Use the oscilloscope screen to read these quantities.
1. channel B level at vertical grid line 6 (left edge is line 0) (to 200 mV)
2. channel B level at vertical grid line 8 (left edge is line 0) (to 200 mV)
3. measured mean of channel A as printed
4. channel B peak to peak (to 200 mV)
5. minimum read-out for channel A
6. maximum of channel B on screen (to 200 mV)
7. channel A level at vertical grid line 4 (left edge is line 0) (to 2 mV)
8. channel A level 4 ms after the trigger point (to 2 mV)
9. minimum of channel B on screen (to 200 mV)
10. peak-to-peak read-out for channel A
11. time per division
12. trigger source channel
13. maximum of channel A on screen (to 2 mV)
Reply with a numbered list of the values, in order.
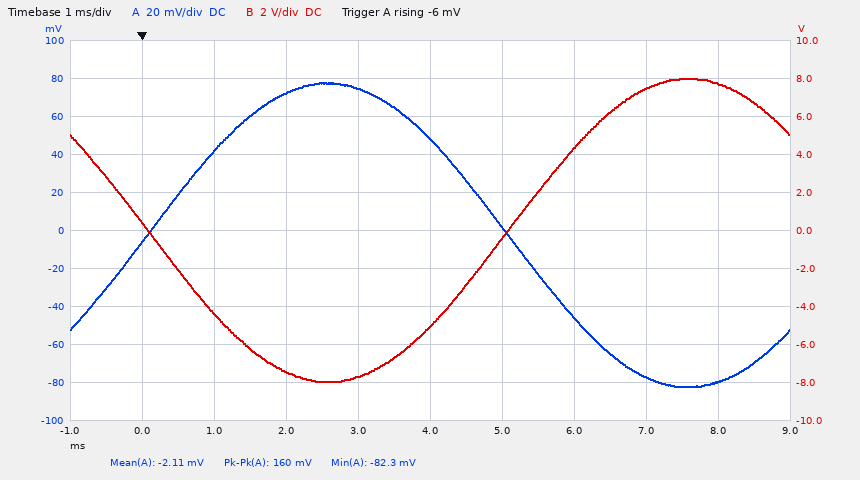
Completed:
1. -400 mV
2. 7.4 V
3. -2.11 mV
4. 16.0 V
5. -82.3 mV
6. 8.0 V
7. 74 mV
8. 48 mV
9. -8.0 V
10. 160 mV
11. 1 ms
12. channel A
13. 78 mV
